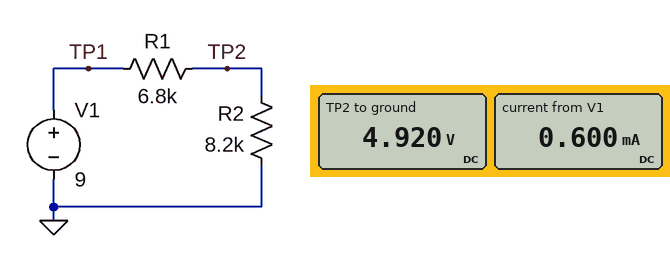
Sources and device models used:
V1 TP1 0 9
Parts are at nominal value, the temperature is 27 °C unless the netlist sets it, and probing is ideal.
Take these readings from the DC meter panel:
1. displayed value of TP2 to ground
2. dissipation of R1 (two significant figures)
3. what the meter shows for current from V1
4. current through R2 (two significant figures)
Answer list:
4.920 V
2.4 mW
0.600 mA
600 µA
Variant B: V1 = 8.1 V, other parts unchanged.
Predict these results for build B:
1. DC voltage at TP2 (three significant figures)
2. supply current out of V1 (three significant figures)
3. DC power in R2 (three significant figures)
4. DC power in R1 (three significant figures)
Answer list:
4.43 V
540 µA
2.39 mW
1.98 mW
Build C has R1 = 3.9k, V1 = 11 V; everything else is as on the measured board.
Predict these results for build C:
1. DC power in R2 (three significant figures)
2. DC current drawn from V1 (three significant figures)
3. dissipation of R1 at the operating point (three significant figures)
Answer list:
6.78 mW
909 µA
3.22 mW
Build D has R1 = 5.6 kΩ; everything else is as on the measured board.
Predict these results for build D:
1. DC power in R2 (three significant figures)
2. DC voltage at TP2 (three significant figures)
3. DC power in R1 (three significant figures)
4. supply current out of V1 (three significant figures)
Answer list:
3.49 mW
5.35 V
2.38 mW
652 µA
